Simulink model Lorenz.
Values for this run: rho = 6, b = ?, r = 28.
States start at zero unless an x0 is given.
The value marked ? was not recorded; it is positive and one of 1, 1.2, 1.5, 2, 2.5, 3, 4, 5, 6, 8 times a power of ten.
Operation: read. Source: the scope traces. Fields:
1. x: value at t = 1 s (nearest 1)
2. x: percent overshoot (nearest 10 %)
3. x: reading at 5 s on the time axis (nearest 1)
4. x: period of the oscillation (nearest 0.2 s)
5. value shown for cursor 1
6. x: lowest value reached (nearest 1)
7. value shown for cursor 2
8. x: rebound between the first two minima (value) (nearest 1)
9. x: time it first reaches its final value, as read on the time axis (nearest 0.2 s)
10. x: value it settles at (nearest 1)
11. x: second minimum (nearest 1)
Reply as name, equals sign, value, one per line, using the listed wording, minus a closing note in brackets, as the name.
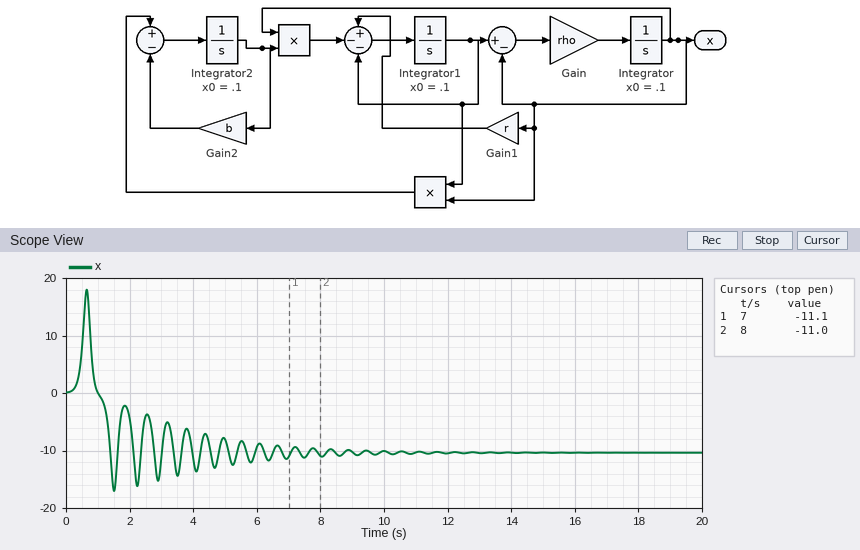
x: value at t = 1 s = 0
x: percent overshoot = 60 %
x: reading at 5 s on the time axis = -8
x: period of the oscillation = 0.8 s
value shown for cursor 1 = -11.1
x: lowest value reached = -17
value shown for cursor 2 = -11.0
x: rebound between the first two minima (value) = -2
x: time it first reaches its final value, as read on the time axis = 1.4 s
x: value it settles at = -10
x: second minimum = -16
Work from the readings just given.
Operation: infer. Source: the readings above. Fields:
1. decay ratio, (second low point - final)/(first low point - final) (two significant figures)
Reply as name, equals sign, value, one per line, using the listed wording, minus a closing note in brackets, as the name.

decay ratio, (second low point - final)/(first low point - final) = 0.86
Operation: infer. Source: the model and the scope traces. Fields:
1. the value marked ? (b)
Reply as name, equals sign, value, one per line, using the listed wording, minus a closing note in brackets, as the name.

the value marked ? = 4
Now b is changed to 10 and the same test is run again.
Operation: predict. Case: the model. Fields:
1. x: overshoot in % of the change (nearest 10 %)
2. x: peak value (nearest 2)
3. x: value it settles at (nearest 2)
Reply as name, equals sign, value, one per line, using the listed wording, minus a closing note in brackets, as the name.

x: overshoot in % of the change = 30 %
x: peak value = 20
x: value it settles at = 16
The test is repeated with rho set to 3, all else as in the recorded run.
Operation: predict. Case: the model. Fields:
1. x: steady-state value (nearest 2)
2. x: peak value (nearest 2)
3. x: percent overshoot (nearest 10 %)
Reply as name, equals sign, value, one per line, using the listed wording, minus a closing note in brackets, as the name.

x: steady-state value = 10
x: peak value = 14
x: percent overshoot = 40 %
